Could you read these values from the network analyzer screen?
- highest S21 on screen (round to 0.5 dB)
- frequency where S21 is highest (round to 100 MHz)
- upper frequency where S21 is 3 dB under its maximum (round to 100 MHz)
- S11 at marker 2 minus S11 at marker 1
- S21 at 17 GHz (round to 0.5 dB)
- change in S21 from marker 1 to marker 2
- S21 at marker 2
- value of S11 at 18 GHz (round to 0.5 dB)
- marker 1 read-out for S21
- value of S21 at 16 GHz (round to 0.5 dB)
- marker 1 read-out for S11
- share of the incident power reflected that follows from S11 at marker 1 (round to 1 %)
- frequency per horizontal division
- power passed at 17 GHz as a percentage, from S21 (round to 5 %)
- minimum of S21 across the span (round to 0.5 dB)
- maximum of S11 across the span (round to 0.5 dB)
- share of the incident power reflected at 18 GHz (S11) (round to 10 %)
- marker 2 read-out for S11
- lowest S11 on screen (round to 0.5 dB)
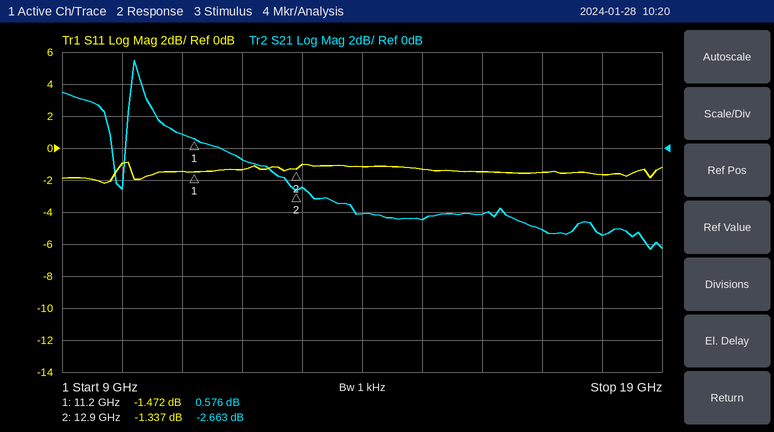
5.5 dB
10.2 GHz
10.5 GHz
0.135 dB
-5.0 dB
-3.239 dB
-2.663 dB
-1.5 dB
0.576 dB
-4.0 dB
-1.472 dB
71 %
1 GHz
30 %
-6.5 dB
-1.0 dB
70 %
-1.337 dB
-2.0 dB
